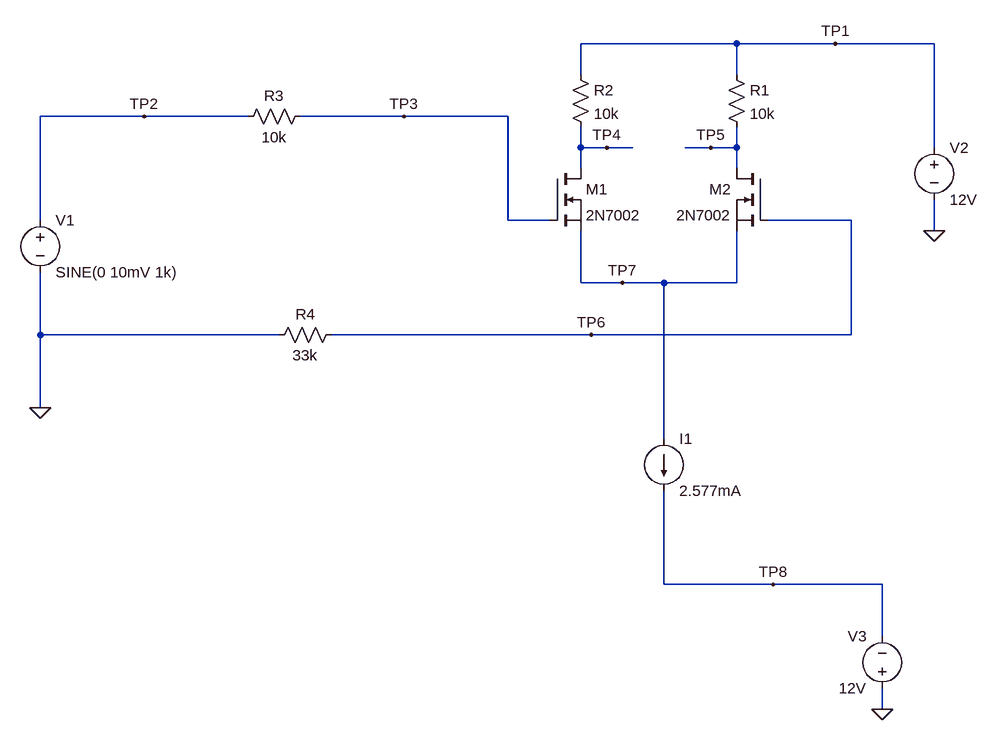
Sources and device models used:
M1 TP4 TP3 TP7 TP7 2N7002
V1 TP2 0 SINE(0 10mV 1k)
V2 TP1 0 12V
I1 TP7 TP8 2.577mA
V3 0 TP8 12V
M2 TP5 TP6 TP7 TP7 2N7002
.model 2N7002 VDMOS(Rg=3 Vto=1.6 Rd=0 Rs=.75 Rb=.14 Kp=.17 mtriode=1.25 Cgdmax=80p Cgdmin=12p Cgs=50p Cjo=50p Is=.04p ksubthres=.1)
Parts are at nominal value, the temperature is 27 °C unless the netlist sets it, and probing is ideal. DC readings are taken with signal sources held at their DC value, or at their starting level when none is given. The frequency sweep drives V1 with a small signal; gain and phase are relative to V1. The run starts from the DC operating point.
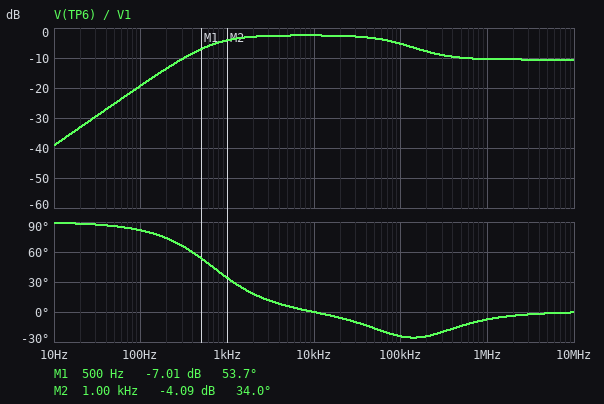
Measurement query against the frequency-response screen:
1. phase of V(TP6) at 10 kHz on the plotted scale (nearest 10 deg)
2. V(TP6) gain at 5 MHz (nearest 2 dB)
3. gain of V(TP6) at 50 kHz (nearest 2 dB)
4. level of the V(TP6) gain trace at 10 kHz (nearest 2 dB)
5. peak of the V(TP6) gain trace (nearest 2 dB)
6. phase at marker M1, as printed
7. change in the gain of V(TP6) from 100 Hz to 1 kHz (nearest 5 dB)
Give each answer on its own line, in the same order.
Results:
0 deg
-10 dB
-4 dB
-2 dB
-2 dB
53.7 deg
15 dB
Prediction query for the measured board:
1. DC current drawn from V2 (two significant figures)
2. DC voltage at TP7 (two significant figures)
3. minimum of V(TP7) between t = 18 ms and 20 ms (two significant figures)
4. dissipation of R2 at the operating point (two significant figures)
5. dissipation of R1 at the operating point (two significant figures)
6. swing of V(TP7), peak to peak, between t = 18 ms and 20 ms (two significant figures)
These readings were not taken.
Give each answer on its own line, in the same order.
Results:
2.6 mA
-1.7 V
-1.7 V
17 mW
17 mW
14 mV
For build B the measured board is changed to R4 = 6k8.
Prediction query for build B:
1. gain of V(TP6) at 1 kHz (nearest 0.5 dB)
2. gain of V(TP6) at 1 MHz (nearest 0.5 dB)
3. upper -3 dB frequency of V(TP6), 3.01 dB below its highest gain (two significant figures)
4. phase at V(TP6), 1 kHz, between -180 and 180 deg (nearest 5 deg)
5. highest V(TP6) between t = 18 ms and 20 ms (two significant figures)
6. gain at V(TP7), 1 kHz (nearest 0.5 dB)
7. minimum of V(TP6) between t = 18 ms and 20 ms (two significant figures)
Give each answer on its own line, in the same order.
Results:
-14.0 dB
-13.0 dB
200 kHz
60 deg
2.0 mV
-6.5 dB
-2.0 mV
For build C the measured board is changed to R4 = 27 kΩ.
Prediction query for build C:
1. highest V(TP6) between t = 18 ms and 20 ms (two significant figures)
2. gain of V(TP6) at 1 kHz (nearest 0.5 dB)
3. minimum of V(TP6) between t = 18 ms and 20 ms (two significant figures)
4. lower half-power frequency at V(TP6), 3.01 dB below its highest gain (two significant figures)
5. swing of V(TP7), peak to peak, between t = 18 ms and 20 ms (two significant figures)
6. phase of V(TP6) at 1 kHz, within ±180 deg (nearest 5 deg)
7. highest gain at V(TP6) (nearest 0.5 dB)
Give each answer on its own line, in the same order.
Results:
5.7 mV
-5.0 dB
-5.6 mV
780 Hz
13 mV
40 deg
-3.0 dB
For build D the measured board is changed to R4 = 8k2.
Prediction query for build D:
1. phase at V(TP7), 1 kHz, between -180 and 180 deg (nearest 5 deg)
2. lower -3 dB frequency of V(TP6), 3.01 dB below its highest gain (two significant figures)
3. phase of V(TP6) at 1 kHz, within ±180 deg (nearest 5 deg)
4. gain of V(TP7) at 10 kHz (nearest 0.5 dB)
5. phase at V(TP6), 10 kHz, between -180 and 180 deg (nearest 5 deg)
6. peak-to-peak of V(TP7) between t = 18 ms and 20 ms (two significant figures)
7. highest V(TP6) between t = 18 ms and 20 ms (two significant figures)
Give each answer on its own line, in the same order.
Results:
-5 deg
1.6 kHz
60 deg
-7.0 dB
5 deg
9.8 mV
2.3 mV
